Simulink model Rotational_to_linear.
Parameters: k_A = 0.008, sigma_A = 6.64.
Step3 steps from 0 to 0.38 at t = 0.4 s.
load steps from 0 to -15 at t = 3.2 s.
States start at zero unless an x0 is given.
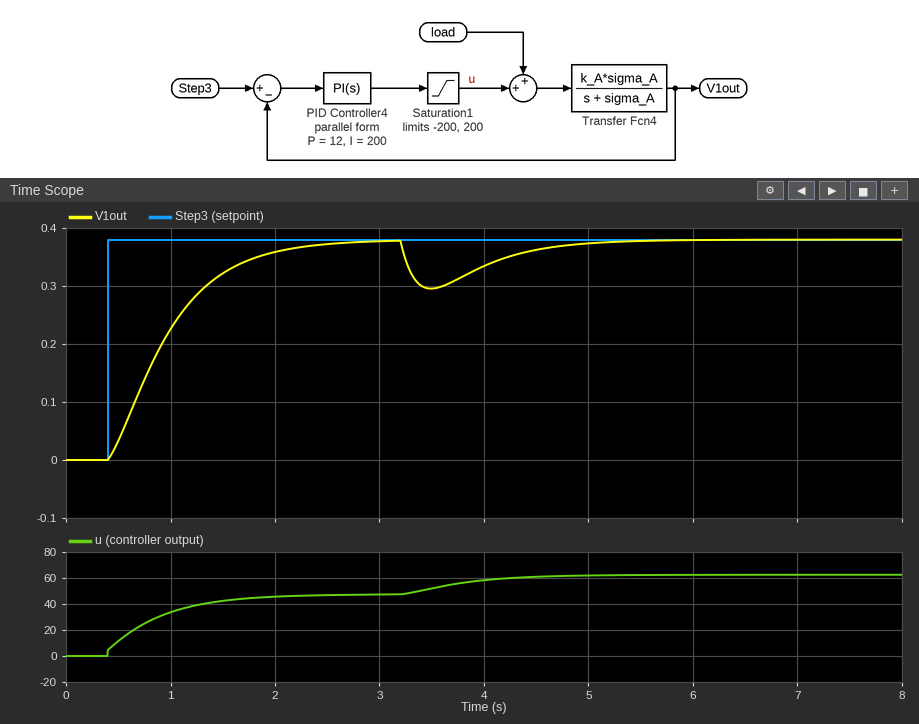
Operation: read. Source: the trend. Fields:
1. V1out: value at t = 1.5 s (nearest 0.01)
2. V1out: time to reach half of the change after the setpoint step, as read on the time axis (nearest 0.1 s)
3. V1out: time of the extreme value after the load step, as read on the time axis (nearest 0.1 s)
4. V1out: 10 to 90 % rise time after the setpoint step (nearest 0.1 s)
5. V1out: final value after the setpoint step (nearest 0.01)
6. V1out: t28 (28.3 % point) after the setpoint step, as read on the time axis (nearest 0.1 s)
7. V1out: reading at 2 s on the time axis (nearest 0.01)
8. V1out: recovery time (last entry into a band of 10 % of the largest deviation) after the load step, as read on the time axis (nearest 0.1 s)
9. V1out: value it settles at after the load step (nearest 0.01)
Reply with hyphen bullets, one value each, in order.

- 0.32
- 0.9 s
- 3.5 s
- 1.2 s
- 0.38
- 0.7 s
- 0.36
- 4.9 s
- 0.38
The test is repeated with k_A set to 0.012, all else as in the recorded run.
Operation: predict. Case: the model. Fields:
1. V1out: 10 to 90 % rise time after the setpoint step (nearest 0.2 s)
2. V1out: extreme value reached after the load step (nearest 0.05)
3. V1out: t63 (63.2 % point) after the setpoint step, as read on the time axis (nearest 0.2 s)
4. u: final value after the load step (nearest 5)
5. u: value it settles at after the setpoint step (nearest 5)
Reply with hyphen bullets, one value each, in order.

- 0.8 s
- 0.25
- 0.8 s
- 45
- 30
